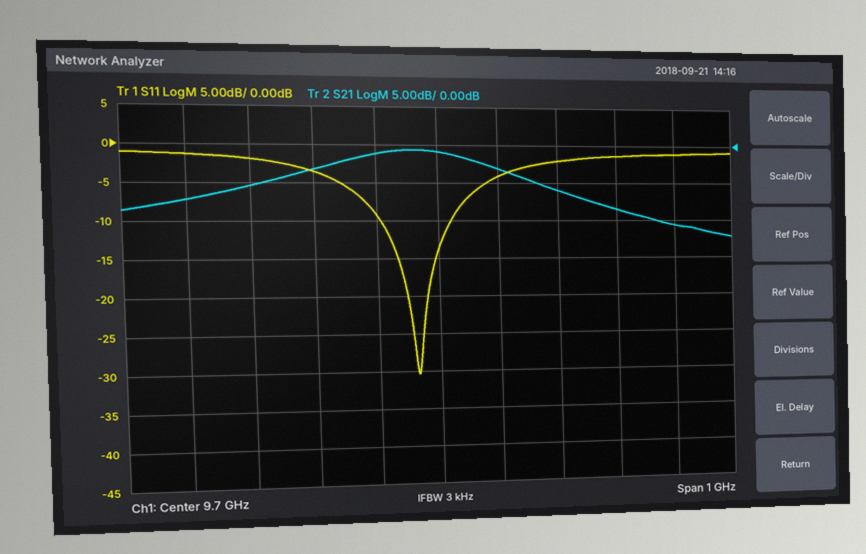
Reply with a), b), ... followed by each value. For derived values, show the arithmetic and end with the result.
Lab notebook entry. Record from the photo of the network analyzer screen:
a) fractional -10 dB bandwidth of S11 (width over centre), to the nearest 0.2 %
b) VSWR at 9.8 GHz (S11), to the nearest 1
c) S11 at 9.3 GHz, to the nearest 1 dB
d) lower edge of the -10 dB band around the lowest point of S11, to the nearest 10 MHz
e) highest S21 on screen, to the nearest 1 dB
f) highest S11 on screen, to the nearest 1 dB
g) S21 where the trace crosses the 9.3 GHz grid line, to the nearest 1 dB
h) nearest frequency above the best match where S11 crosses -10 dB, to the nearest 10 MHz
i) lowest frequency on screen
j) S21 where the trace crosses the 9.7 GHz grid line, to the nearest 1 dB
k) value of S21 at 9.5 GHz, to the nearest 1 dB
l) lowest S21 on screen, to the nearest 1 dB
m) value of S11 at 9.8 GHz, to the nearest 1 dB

a) 110 MHz / 9.665 GHz ≈ 1.14 %, so 1.2 % to the nearest 0.2 %
b) |Γ| = 10^(-4/20) = 0.6310; VSWR = (1 + 0.6310)/(1 − 0.6310) ≈ 4
c) -1 dB
d) 9.61 GHz
e) -1 dB
f) -1 dB
g) -7 dB
h) 9.72 GHz
i) 9.2 GHz
j) -1 dB
k) -3 dB
l) -12 dB
m) -4 dB
